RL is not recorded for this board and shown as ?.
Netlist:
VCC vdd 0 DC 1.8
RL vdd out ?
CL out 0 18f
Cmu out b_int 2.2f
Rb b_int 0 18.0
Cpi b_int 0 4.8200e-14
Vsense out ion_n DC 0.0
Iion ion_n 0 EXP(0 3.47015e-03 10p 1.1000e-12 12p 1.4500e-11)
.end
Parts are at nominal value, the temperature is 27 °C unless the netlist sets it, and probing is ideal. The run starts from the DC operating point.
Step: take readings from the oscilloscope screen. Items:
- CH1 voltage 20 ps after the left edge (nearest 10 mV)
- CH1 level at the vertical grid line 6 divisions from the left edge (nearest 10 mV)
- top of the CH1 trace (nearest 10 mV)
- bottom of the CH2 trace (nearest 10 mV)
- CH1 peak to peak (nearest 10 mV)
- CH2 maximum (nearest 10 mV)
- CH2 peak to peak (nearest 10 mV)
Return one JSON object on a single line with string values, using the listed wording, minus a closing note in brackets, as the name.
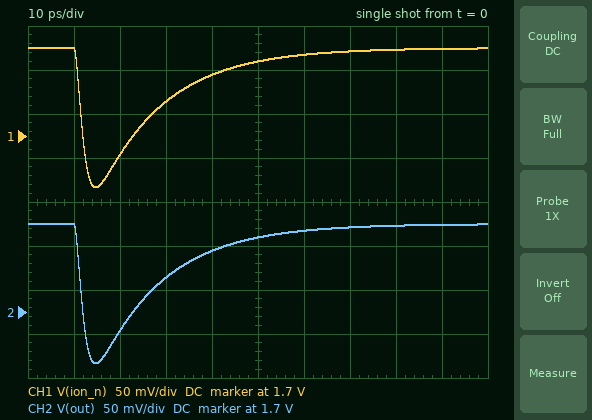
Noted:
{"CH1 voltage 20 ps after the left edge": "1.68 V", "CH1 level at the vertical grid line 6 divisions from the left edge": "1.79 V", "top of the CH1 trace": "1.80 V", "bottom of the CH2 trace": "1.64 V", "CH1 peak to peak": "160 mV", "CH2 maximum": "1.80 V", "CH2 peak to peak": "160 mV"}
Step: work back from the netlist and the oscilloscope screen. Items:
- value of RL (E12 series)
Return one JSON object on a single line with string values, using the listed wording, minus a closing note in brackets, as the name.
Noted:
{"value of RL": "56 Ω"}
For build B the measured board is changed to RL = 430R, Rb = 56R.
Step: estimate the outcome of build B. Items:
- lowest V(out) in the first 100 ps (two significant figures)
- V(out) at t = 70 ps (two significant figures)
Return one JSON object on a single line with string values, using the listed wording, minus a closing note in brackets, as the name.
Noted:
{"lowest V(out) in the first 100 ps": "1.1 V", "V(out) at t = 70 ps": "1.7 V"}
